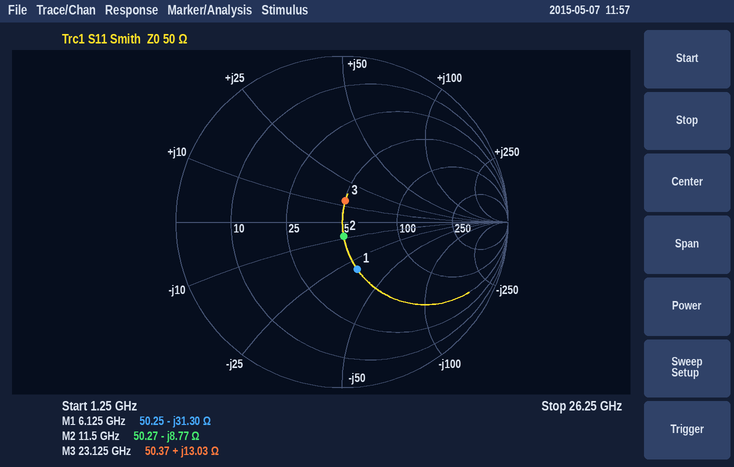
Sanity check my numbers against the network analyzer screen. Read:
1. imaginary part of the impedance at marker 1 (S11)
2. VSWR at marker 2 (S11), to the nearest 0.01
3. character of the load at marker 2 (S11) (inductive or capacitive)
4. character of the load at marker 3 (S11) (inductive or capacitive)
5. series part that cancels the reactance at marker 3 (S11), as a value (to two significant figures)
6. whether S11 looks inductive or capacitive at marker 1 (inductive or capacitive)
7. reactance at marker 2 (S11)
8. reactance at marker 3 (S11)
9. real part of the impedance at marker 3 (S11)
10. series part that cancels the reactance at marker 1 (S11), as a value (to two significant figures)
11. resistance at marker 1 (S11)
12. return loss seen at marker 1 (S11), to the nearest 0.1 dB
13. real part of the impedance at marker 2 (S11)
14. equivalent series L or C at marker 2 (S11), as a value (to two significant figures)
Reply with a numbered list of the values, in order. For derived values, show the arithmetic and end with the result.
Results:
1. -31.30 Ω
2. 1.19
3. capacitive
4. inductive
5. C = 1/(2π × 23.125 GHz × 13.03 Ω) ≈ 528 fF, so 530 fF to two significant figures
6. capacitive
7. -8.77 Ω
8. +13.03 Ω
9. 50.37 Ω
10. L = 31.3 Ω/(2π × 6.125 GHz) ≈ 813 pH, so 810 pH to two significant figures
11. 50.25 Ω
12. 10.5 dB
13. 50.27 Ω
14. C = 1/(2π × 11.5 GHz × 8.77 Ω) ≈ 1.6 pF
